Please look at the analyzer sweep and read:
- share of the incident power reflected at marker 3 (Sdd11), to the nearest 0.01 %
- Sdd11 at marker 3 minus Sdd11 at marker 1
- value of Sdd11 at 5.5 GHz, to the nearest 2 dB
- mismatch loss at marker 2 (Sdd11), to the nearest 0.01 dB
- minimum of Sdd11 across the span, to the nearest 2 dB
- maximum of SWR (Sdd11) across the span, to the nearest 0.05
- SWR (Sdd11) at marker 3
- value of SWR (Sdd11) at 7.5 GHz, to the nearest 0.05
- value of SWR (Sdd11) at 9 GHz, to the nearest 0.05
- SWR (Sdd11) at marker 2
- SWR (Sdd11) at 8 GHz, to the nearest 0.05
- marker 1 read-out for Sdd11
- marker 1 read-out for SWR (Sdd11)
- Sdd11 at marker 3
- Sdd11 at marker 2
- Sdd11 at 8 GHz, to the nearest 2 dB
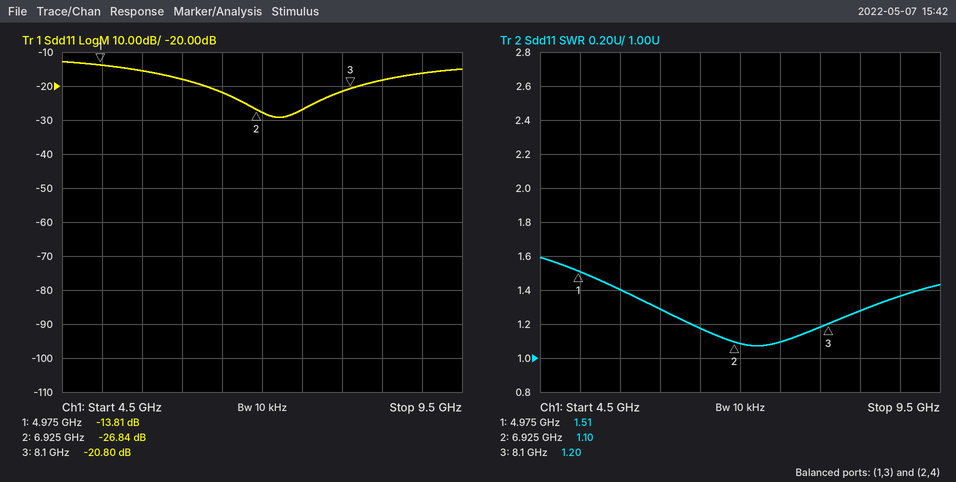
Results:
0.83 %
-6.99 dB
-16 dB
0.01 dB
-30 dB
1.60
1.20
1.10
1.35
1.10
1.20
-13.81 dB
1.51
-20.80 dB
-26.84 dB
-22 dB
